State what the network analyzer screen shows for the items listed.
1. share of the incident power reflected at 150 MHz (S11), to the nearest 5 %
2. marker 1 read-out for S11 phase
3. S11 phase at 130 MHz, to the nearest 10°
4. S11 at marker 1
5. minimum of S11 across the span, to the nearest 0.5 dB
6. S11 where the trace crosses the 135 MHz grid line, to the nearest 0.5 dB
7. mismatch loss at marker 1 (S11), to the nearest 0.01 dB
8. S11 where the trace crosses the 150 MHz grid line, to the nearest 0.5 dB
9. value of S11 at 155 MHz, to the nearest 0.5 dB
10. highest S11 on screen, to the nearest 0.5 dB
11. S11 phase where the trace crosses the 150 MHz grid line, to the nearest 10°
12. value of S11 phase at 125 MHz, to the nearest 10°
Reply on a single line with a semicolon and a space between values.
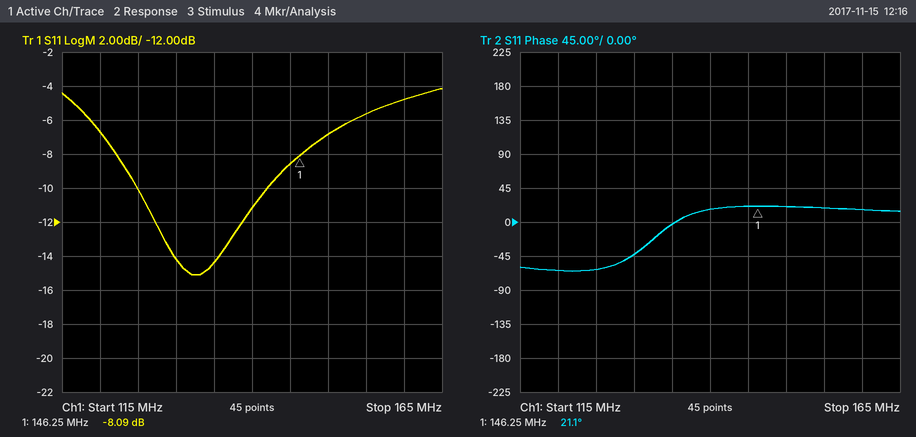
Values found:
20 %; 21.1°; -40°; -8.09 dB; -15.0 dB; -14.5 dB; 0.73 dB; -7.0 dB; -5.5 dB; -4.0 dB; 20°; -60°
